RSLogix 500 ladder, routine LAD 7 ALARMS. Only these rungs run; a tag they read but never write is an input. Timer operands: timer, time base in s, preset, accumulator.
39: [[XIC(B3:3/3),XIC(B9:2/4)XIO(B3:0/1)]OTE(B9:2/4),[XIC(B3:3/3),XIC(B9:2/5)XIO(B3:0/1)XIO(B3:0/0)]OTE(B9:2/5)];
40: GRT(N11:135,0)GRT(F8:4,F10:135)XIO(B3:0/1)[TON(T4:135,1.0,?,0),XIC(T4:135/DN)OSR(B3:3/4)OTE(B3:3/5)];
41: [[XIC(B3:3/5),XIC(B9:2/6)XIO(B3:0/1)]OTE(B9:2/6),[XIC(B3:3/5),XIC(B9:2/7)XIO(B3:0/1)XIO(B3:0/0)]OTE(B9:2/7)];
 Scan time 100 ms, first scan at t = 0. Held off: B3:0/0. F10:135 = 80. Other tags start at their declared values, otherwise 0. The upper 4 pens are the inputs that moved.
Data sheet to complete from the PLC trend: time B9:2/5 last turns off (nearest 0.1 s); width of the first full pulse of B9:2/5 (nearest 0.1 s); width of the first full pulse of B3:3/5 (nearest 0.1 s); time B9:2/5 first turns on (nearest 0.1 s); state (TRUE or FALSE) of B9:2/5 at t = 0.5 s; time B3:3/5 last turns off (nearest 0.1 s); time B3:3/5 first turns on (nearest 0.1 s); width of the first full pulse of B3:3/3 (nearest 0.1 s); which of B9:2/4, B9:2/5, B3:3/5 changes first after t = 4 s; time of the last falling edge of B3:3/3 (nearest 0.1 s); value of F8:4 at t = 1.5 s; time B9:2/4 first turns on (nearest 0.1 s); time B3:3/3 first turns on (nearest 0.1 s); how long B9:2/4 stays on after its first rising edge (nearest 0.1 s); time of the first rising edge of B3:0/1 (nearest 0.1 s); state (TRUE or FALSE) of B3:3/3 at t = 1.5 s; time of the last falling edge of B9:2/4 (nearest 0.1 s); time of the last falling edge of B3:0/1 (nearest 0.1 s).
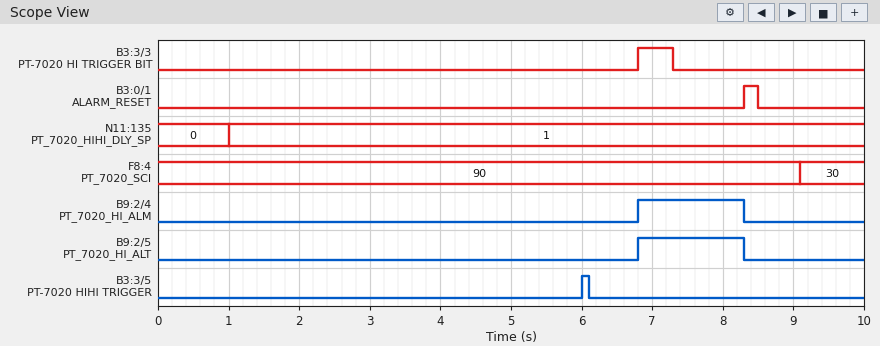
8.3 s
1.5 s
0.1 s
6.8 s
FALSE
6.1 s
6.0 s
0.5 s
B3:3/5
7.3 s
90
6.8 s
6.8 s
1.5 s
8.3 s
FALSE
8.3 s
8.5 s
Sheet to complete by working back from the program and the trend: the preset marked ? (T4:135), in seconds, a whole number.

5 s
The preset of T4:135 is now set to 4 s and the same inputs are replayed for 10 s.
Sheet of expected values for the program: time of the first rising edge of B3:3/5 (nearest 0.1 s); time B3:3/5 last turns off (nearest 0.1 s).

5.0 s
5.1 s
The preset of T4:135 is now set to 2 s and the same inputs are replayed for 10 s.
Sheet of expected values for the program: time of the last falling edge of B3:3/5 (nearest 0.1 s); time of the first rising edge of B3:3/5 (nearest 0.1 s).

3.1 s
3.0 s
